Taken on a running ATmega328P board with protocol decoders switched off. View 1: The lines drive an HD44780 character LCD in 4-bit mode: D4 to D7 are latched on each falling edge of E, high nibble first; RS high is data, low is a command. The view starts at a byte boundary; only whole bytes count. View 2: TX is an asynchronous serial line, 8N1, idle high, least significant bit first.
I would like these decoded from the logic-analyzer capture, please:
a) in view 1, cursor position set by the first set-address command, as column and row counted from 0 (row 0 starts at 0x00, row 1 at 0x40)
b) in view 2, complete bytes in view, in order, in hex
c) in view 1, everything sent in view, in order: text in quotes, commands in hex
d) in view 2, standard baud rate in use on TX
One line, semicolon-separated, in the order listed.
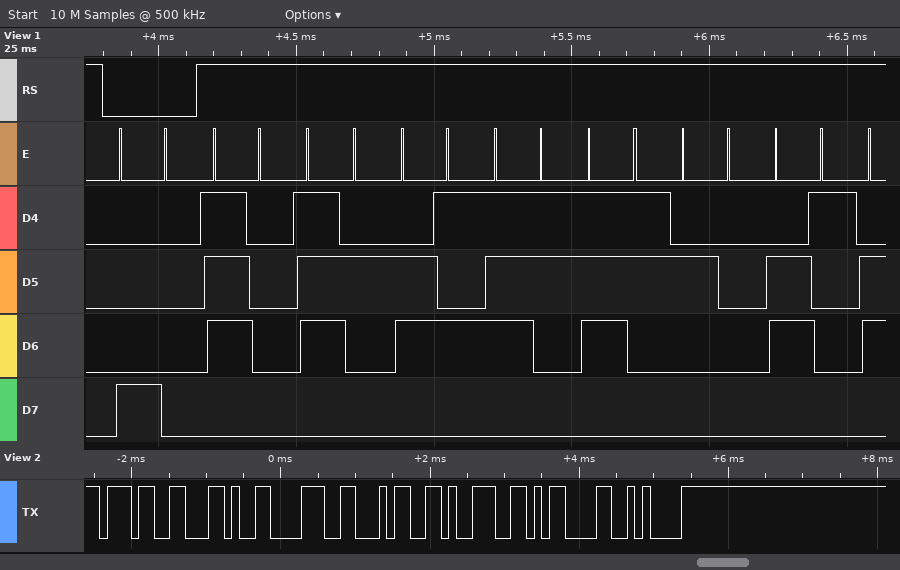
column 0, row 0; 37 2C 38 34 39 0D 0A; 0x80 "press a"; 9600 baud
